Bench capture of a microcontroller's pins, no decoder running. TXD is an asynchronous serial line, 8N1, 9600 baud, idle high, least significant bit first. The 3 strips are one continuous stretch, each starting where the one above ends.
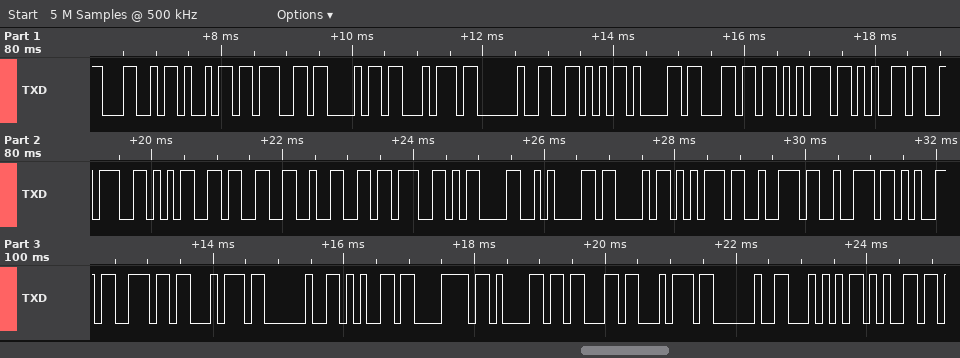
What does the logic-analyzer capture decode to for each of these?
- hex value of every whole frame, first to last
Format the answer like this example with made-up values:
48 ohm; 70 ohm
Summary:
4C 69 67 68 74 20 56 61 6C 75 65 3A 35 33 32 3B 0D 0A 43 75 72 72 65 6E 74 20 65 78 61 63 74 20 54 65
